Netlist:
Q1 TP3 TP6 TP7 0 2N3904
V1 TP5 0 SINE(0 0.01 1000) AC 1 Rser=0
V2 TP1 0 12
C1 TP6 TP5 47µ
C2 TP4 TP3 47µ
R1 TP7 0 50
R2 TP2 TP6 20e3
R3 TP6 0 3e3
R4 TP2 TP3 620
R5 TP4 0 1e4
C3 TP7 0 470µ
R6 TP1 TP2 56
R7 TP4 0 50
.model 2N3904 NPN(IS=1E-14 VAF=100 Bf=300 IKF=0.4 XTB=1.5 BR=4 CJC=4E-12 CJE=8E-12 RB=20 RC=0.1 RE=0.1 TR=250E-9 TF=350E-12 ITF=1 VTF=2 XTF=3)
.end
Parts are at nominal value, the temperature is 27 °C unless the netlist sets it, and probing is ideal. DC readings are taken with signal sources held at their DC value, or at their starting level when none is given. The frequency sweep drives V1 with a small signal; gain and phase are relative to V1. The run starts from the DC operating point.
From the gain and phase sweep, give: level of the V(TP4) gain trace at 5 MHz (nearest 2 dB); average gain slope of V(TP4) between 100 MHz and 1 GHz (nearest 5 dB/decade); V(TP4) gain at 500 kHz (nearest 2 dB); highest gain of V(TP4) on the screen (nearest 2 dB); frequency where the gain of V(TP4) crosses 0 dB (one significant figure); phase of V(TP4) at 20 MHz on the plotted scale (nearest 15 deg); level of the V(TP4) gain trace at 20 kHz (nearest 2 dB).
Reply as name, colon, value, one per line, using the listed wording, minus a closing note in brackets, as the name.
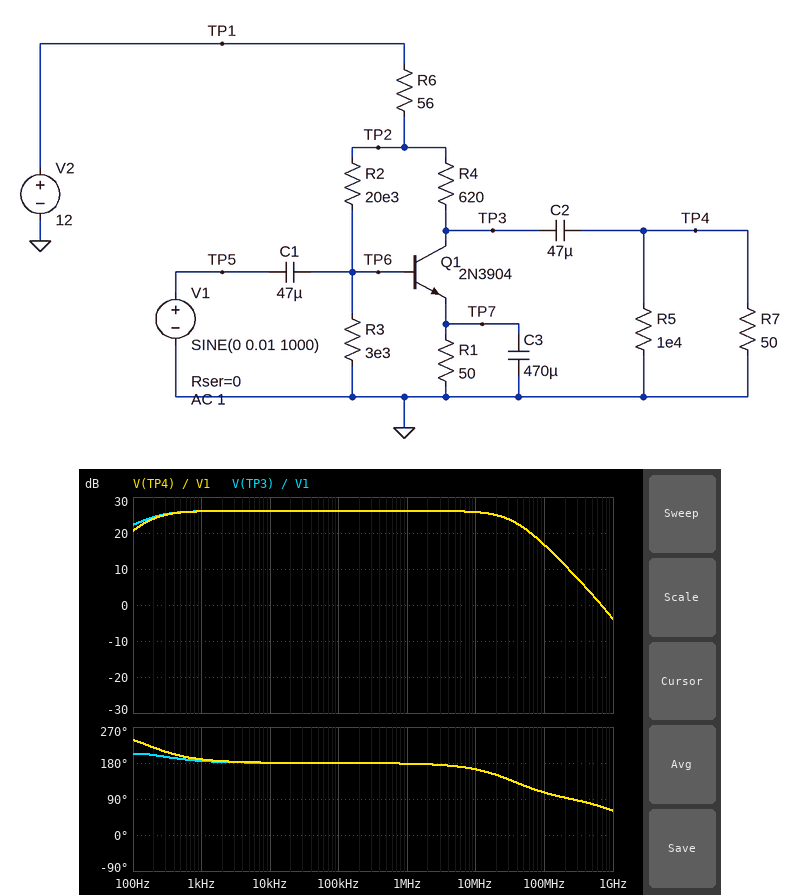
level of the V(TP4) gain trace at 5 MHz: 26 dB
average gain slope of V(TP4) between 100 MHz and 1 GHz: -20 dB/decade
V(TP4) gain at 500 kHz: 26 dB
highest gain of V(TP4) on the screen: 26 dB
frequency where the gain of V(TP4) crosses 0 dB: 700 MHz
phase of V(TP4) at 20 MHz on the plotted scale: 150 deg
level of the V(TP4) gain trace at 20 kHz: 26 dB
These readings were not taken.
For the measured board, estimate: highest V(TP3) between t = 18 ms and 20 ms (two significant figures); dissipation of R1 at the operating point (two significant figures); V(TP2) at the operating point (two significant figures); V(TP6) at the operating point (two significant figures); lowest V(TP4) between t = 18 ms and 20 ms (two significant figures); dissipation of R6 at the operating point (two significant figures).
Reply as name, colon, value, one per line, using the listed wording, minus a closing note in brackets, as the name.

highest V(TP3) between t = 18 ms and 20 ms: 3.6 V
dissipation of R1 at the operating point: 8.1 mW
V(TP2) at the operating point: 11 V
V(TP6) at the operating point: 1.4 V
lowest V(TP4) between t = 18 ms and 20 ms: -210 mV
dissipation of R6 at the operating point: 9.7 mW
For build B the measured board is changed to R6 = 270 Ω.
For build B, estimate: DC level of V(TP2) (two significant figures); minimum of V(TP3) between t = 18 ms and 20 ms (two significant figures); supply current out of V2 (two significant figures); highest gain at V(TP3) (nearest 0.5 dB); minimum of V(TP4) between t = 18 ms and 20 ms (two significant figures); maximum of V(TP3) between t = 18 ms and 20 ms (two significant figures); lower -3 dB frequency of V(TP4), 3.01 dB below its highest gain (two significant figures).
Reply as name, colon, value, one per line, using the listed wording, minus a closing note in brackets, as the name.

DC level of V(TP2): 9.5 V
minimum of V(TP3) between t = 18 ms and 20 ms: 3.8 V
supply current out of V2: 9.3 mA
highest gain at V(TP3): 23.5 dB
minimum of V(TP4) between t = 18 ms and 20 ms: -160 mV
maximum of V(TP3) between t = 18 ms and 20 ms: 4.1 V
lower -3 dB frequency of V(TP4), 3.01 dB below its highest gain: 120 Hz
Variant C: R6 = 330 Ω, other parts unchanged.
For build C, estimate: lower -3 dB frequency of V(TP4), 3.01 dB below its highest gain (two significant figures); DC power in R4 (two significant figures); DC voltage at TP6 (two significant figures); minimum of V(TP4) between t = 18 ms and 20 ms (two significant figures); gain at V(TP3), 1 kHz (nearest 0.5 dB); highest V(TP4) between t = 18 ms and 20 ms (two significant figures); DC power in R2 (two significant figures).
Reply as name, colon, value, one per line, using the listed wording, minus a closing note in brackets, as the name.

lower -3 dB frequency of V(TP4), 3.01 dB below its highest gain: 110 Hz
DC power in R4: 42 mW
DC voltage at TP6: 1.1 V
minimum of V(TP4) between t = 18 ms and 20 ms: -150 mV
gain at V(TP3), 1 kHz: 23.0 dB
highest V(TP4) between t = 18 ms and 20 ms: 130 mV
DC power in R2: 3.2 mW
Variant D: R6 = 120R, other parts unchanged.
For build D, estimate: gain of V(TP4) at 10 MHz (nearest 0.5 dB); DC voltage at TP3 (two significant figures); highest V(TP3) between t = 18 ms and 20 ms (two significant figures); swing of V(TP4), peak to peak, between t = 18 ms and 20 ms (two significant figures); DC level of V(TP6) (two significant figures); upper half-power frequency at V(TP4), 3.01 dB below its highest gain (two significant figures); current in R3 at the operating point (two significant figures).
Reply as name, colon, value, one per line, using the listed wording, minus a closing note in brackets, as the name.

gain of V(TP4) at 10 MHz: 25.0 dB
DC voltage at TP3: 3.6 V
highest V(TP3) between t = 18 ms and 20 ms: 3.8 V
swing of V(TP4), peak to peak, between t = 18 ms and 20 ms: 360 mV
DC level of V(TP6): 1.3 V
upper half-power frequency at V(TP4), 3.01 dB below its highest gain: 40 MHz
current in R3 at the operating point: 430 µA
